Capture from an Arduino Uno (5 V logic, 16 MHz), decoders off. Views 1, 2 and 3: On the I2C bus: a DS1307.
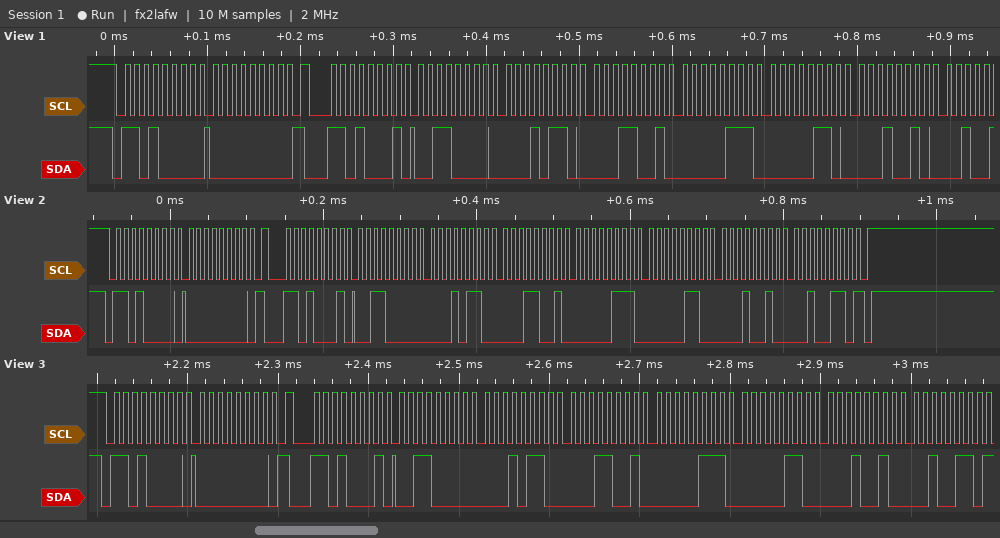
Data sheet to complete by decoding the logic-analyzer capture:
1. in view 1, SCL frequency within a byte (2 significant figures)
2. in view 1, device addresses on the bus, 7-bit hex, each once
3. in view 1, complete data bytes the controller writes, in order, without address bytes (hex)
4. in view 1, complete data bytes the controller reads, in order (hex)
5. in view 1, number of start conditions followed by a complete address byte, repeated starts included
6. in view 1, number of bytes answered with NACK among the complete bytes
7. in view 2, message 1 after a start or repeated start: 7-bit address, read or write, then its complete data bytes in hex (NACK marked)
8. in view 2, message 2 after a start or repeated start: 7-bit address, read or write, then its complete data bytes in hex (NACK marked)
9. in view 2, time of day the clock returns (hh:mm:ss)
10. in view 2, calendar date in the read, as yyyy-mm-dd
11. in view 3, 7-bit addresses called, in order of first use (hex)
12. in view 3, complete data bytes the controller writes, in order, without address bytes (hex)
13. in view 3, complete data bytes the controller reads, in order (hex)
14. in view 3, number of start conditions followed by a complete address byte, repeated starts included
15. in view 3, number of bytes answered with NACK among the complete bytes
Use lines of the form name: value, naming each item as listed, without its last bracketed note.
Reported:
in view 1, SCL frequency within a byte: 100 kHz
in view 1, device addresses on the bus, 7-bit hex, each once: 0x68
in view 1, complete data bytes the controller writes, in order, without address bytes: 00
in view 1, complete data bytes the controller reads, in order: 30 16 19 07 06 12
in view 1, number of start conditions followed by a complete address byte, repeated starts included: 2
in view 1, number of bytes answered with NACK among the complete bytes: 0
in view 2, message 1 after a start or repeated start: 7-bit address, read or write, then its complete data bytes in hex: 0x68 write: 00
in view 2, message 2 after a start or repeated start: 7-bit address, read or write, then its complete data bytes in hex: 0x68 read: 30 16 19 07 06 12 26 NACK
in view 2, time of day the clock returns: 19:16:30
in view 2, calendar date in the read, as yyyy-mm-dd: 2026-12-06
in view 3, 7-bit addresses called, in order of first use: 0x68
in view 3, complete data bytes the controller writes, in order, without address bytes: 00
in view 3, complete data bytes the controller reads, in order: 30 16 19 07 06 12 26
in view 3, number of start conditions followed by a complete address byte, repeated starts included: 2
in view 3, number of bytes answered with NACK among the complete bytes: 1
